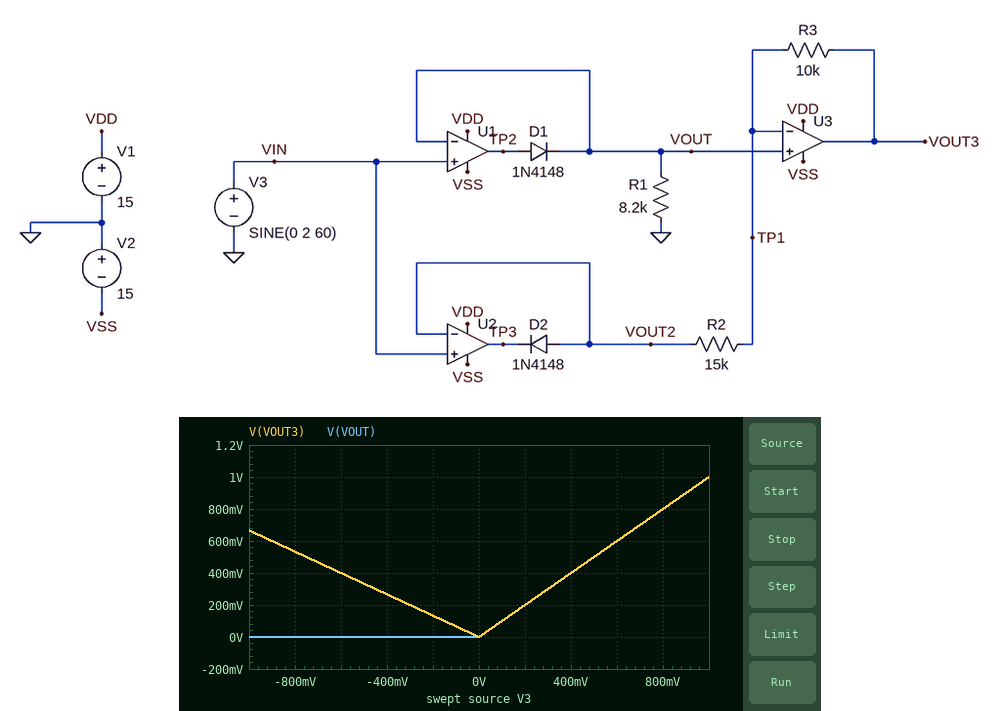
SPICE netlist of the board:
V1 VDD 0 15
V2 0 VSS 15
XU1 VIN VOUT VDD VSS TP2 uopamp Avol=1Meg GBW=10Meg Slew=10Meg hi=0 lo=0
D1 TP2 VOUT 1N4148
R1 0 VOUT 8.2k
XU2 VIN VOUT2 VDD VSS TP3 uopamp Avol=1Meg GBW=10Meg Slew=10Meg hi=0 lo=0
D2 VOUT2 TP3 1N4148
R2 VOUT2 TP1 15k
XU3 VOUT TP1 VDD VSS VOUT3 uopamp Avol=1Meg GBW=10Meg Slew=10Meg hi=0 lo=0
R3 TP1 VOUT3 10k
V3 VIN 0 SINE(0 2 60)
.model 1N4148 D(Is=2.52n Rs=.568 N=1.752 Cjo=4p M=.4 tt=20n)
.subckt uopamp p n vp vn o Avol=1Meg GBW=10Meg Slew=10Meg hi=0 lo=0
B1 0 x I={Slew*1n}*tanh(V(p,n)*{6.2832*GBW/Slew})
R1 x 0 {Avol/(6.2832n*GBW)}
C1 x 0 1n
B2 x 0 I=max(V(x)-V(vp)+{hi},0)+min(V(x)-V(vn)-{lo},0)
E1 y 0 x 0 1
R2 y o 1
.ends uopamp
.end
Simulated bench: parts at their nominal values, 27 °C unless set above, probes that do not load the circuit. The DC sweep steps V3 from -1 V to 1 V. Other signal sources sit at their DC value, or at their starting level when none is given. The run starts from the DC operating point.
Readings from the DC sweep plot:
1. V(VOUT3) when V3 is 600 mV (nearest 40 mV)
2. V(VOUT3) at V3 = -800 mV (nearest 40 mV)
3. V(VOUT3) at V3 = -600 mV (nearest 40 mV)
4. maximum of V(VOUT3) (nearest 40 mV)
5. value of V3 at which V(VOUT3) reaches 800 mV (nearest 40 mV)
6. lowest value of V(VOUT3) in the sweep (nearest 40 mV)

600 mV
520 mV
400 mV
1.00 V
800 mV
0 V
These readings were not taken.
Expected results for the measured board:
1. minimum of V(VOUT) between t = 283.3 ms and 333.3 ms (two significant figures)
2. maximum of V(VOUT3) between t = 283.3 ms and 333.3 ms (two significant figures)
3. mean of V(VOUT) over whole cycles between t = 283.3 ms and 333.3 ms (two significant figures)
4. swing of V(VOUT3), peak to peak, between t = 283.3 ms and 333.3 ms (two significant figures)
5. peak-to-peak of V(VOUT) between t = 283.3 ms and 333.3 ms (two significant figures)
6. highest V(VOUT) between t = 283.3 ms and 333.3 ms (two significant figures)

-11 mV
2.0 V
640 mV
2.0 V
2.0 V
2.0 V
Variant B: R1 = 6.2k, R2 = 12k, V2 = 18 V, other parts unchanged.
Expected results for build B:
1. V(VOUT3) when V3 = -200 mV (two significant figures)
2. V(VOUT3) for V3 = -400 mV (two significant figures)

170 mV
330 mV
